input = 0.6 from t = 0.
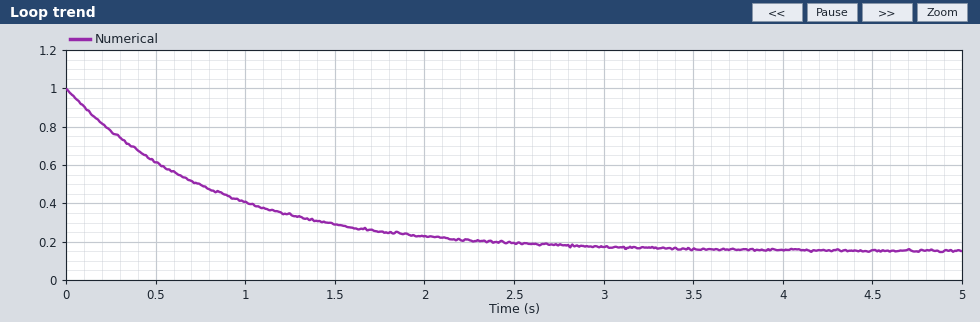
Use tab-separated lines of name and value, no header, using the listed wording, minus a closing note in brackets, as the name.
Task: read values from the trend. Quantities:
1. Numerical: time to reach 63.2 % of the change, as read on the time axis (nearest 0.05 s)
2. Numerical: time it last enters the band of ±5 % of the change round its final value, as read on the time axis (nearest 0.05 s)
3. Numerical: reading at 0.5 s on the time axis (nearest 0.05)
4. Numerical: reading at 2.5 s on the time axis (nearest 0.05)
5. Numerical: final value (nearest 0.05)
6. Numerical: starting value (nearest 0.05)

Numerical: time to reach 63.2 % of the change, as read on the time axis	0.85 s
Numerical: time it last enters the band of ±5 % of the change round its final value, as read on the time axis	2.50 s
Numerical: reading at 0.5 s on the time axis	0.60
Numerical: reading at 2.5 s on the time axis	0.20
Numerical: final value	0.15
Numerical: starting value	1.00
